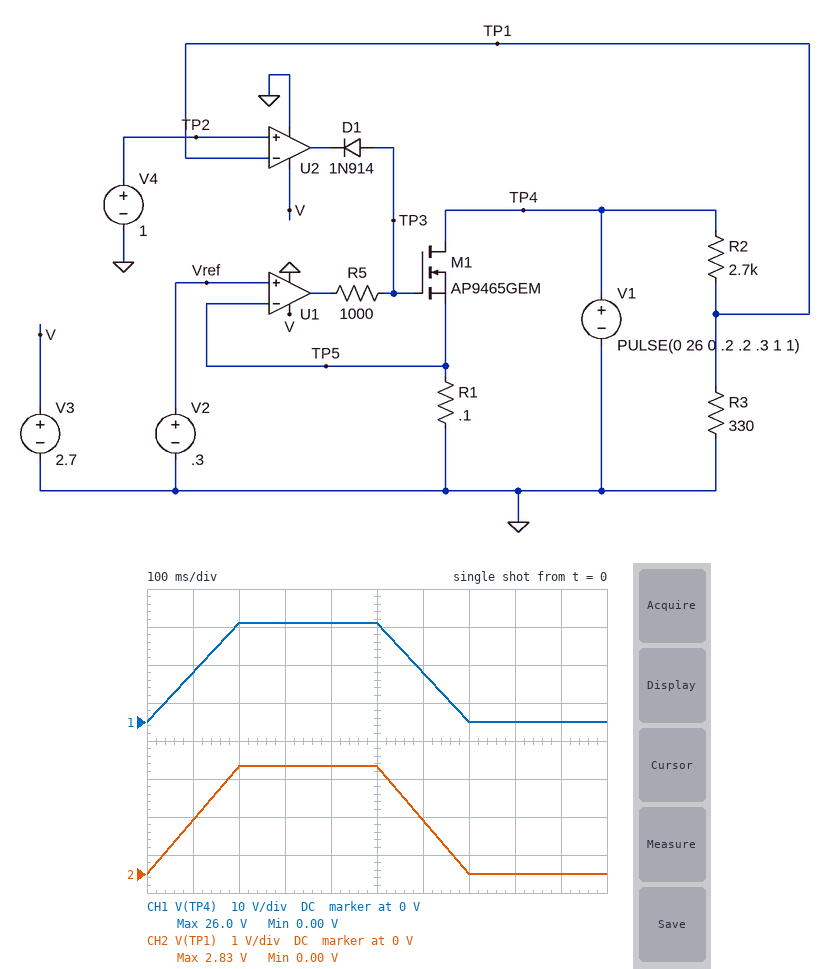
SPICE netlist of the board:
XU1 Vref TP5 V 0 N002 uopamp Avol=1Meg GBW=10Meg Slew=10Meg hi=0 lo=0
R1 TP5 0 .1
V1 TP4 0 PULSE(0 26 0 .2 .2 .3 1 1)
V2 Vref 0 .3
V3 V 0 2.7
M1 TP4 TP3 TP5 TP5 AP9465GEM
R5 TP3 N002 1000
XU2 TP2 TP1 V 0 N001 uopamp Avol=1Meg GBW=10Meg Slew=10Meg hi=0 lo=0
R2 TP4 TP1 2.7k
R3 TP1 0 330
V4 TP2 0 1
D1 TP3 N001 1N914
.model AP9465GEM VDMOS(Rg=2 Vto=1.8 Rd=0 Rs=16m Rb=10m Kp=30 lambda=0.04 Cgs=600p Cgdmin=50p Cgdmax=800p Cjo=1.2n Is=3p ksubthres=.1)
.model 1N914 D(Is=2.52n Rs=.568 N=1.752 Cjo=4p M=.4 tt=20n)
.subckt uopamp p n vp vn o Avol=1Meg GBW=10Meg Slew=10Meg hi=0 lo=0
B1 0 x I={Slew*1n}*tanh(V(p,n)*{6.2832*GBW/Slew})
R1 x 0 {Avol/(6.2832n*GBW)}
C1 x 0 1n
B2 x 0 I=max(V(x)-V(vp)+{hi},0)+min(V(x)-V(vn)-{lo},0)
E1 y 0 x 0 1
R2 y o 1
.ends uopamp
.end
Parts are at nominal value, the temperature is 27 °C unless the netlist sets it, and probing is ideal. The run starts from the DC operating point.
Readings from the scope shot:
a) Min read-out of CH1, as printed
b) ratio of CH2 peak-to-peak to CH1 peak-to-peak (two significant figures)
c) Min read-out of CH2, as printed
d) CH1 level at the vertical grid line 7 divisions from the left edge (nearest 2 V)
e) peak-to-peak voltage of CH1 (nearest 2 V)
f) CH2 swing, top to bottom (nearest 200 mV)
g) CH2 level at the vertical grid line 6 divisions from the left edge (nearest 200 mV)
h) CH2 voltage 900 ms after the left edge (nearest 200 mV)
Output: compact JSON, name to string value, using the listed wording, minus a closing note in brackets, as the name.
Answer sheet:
{"Min read-out of CH1, as printed": "0.00 V", "ratio of CH2 peak-to-peak to CH1 peak-to-peak": "0.11", "Min read-out of CH2, as printed": "0.00 V", "CH1 level at the vertical grid line 7 divisions from the left edge": "0 V", "peak-to-peak voltage of CH1": "26 V", "CH2 swing, top to bottom": "2.8 V", "CH2 level at the vertical grid line 6 divisions from the left edge": "1.4 V", "CH2 voltage 900 ms after the left edge": "0 V"}
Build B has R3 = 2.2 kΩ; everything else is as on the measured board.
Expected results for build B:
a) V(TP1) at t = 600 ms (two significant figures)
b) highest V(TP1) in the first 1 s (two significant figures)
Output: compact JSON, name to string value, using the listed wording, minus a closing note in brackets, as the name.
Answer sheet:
{"V(TP1) at t = 600 ms": "5.8 V", "highest V(TP1) in the first 1 s": "12 V"}
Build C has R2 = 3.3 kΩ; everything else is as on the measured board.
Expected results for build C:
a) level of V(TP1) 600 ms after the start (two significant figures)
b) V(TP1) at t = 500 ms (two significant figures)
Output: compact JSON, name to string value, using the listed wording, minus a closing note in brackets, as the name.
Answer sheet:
{"level of V(TP1) 600 ms after the start": "1.2 V", "V(TP1) at t = 500 ms": "2.4 V"}
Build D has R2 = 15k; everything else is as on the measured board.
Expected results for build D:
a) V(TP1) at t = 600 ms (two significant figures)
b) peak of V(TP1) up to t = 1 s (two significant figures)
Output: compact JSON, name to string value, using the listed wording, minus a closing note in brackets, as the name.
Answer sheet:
{"V(TP1) at t = 600 ms": "280 mV", "peak of V(TP1) up to t = 1 s": "560 mV"}
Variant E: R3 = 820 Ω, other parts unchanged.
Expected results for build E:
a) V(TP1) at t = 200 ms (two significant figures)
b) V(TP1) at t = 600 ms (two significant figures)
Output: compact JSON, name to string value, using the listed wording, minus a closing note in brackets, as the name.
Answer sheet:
{"V(TP1) at t = 200 ms": "6.1 V", "V(TP1) at t = 600 ms": "3.0 V"}
